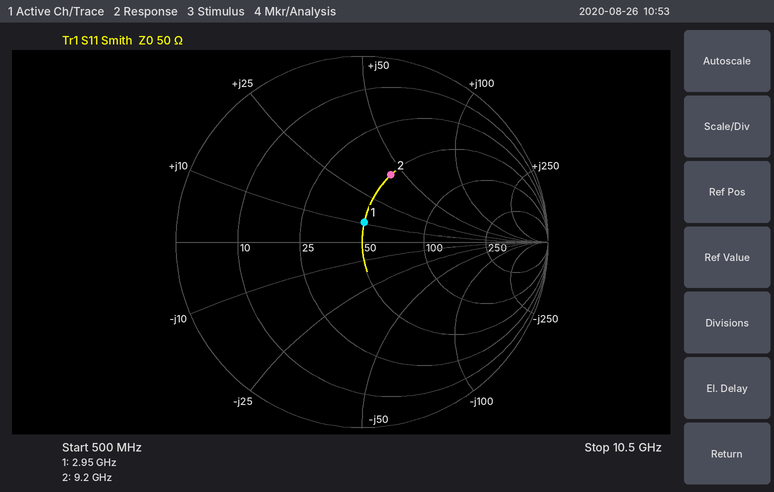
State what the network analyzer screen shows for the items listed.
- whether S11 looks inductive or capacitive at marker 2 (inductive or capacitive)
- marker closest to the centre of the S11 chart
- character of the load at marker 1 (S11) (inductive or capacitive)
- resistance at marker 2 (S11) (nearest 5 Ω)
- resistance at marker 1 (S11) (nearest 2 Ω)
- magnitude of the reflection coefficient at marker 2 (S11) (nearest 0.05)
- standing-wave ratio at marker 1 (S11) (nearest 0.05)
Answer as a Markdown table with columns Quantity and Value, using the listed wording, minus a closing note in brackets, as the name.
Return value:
| Quantity | Value |
|---|---|
| whether S11 looks inductive or capacitive at marker 2 | inductive |
| marker closest to the centre of the S11 chart | marker 1 |
| character of the load at marker 1 (S11) | inductive |
| resistance at marker 2 (S11) | 50 Ω |
| resistance at marker 1 (S11) | 50 Ω |
| magnitude of the reflection coefficient at marker 2 (S11) | 0.40 |
| standing-wave ratio at marker 1 (S11) | 1.25 |
